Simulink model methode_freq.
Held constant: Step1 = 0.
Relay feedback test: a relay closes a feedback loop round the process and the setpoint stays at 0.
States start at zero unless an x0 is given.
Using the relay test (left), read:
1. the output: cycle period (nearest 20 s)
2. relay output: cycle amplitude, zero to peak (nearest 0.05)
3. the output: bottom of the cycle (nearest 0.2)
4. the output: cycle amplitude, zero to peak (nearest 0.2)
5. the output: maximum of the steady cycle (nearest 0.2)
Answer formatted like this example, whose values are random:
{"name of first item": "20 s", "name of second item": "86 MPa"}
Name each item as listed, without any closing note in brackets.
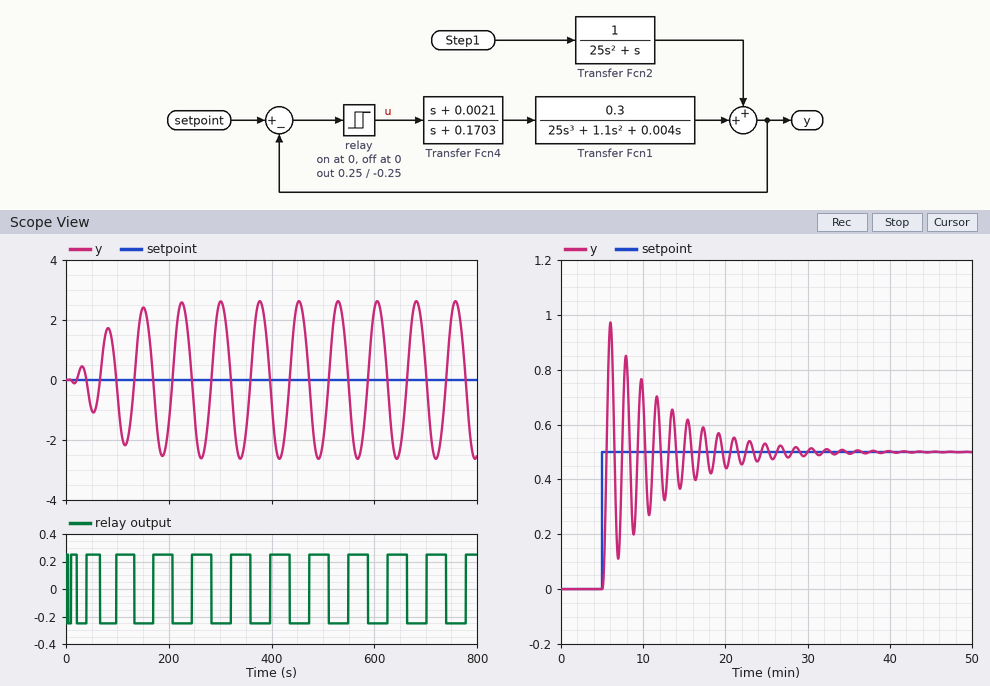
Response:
{"the output: cycle period": "80 s", "relay output: cycle amplitude, zero to peak": "0.25", "the output: bottom of the cycle": "-2.6", "the output: cycle amplitude, zero to peak": "2.6", "the output: maximum of the steady cycle": "2.6"}
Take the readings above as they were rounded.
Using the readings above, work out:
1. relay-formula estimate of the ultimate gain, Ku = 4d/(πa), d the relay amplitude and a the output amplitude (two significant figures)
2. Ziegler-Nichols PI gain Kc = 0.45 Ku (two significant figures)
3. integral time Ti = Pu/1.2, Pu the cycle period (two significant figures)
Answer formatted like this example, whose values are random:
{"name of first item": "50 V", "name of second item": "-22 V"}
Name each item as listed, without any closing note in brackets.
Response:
{"relay-formula estimate of the ultimate gain, Ku = 4d/(πa), d the relay amplitude and a the output amplitude": "0.12", "Ziegler-Nichols PI gain Kc = 0.45 Ku": "0.054", "integral time Ti = Pu/1.2, Pu the cycle period": "67 s"}
